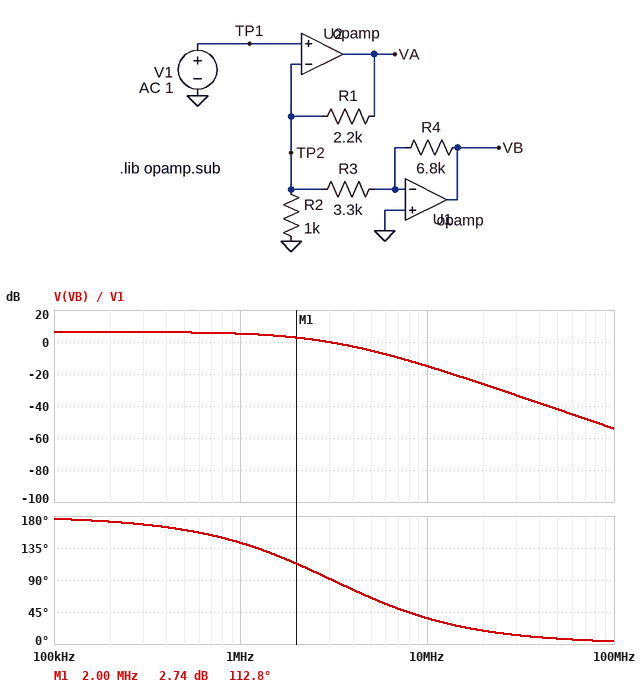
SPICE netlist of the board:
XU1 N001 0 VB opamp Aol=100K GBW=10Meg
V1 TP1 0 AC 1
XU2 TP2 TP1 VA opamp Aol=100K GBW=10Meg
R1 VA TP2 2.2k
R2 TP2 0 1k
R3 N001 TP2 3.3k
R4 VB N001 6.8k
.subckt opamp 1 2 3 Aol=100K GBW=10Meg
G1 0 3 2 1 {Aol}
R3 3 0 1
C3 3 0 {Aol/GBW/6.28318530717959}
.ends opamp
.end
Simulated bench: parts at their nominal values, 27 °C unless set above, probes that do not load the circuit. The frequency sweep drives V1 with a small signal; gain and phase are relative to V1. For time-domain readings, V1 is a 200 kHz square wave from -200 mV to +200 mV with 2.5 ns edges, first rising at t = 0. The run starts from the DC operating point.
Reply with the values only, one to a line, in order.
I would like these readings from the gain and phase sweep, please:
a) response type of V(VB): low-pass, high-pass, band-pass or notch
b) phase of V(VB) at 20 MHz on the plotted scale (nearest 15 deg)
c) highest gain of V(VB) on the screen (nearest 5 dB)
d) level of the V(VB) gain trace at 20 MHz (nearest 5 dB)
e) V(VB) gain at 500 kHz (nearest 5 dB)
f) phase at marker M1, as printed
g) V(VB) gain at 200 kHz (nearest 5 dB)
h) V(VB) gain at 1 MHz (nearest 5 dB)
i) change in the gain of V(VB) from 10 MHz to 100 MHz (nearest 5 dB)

low-pass
15 deg
5 dB
-25 dB
5 dB
112.8 deg
5 dB
5 dB
-40 dB
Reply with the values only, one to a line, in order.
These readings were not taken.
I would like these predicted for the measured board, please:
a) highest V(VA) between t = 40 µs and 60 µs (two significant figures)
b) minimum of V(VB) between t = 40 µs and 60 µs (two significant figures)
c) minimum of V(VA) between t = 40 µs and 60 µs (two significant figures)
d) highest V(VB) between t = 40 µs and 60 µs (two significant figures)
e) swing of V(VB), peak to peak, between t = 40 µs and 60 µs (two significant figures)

770 mV
-410 mV
-770 mV
410 mV
820 mV
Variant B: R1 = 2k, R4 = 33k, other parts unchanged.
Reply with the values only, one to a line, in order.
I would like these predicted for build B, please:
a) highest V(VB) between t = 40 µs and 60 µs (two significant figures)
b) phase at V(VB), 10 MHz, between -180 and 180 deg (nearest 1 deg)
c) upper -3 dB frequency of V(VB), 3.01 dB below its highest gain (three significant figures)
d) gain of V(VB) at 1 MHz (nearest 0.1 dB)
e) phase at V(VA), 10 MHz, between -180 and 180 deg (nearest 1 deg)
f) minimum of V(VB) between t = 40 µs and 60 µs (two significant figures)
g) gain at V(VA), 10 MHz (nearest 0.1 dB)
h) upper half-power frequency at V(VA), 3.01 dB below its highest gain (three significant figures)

2.0 V
24 deg
807 kHz
15.9 dB
-72 deg
-2.0 V
-0.5 dB
2.11 MHz
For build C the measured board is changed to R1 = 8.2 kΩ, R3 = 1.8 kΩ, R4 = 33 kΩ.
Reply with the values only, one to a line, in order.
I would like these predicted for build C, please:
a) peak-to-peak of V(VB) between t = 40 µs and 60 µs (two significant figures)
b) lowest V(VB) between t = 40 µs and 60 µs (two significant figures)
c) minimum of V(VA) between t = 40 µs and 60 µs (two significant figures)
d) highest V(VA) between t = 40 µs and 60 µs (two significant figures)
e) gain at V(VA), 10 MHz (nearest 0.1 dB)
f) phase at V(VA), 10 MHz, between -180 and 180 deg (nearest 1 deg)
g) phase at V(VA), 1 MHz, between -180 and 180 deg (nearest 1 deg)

7.3 V
-3.6 V
-2.7 V
2.7 V
-0.1 dB
-84 deg
-51 deg
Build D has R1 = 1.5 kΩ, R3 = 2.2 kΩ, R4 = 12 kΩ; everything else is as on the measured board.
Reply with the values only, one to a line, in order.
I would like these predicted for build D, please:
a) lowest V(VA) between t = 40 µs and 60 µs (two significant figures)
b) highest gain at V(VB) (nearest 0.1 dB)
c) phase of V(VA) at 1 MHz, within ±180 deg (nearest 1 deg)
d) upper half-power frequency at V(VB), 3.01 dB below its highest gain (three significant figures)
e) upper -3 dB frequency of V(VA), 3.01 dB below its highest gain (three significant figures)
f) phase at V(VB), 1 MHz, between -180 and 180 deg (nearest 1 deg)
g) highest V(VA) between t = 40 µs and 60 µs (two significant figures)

-640 mV
14.7 dB
-21 deg
1.25 MHz
2.32 MHz
131 deg
640 mV
